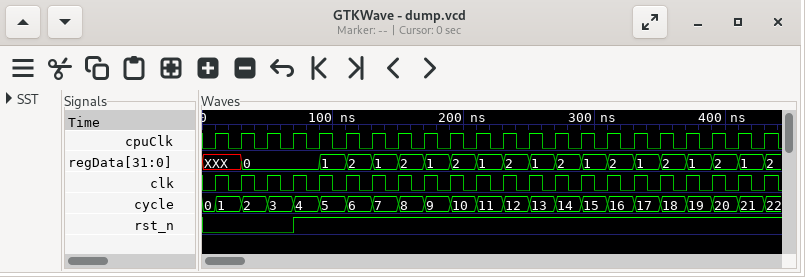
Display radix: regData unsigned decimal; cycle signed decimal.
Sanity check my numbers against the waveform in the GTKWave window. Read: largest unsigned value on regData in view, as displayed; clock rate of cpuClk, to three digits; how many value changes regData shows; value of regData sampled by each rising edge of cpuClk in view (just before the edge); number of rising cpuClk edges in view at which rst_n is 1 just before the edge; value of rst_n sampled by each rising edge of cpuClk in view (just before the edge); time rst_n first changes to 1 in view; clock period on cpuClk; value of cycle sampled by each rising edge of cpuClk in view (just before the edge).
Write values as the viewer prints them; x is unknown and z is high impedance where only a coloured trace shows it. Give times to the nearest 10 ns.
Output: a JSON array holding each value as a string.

["2", "50.0 MHz", "19", "XXX, XXX, 0, 0, 0, 1, 2, 1, 2, 1, 2, 1, 2, 1, 2, 1, 2, 1, 2, 1, 2, 1", "18", "0 0 0 0 1 1 1 1 1 1 1 1 1 1 1 1 1 1 1 1 1 1", "70 ns", "20 ns", "0, 1, 2, 3, 4, 5, 6, 7, 8, 9, 10, 11, 12, 13, 14, 15, 16, 17, 18, 19, 20, 21"]
